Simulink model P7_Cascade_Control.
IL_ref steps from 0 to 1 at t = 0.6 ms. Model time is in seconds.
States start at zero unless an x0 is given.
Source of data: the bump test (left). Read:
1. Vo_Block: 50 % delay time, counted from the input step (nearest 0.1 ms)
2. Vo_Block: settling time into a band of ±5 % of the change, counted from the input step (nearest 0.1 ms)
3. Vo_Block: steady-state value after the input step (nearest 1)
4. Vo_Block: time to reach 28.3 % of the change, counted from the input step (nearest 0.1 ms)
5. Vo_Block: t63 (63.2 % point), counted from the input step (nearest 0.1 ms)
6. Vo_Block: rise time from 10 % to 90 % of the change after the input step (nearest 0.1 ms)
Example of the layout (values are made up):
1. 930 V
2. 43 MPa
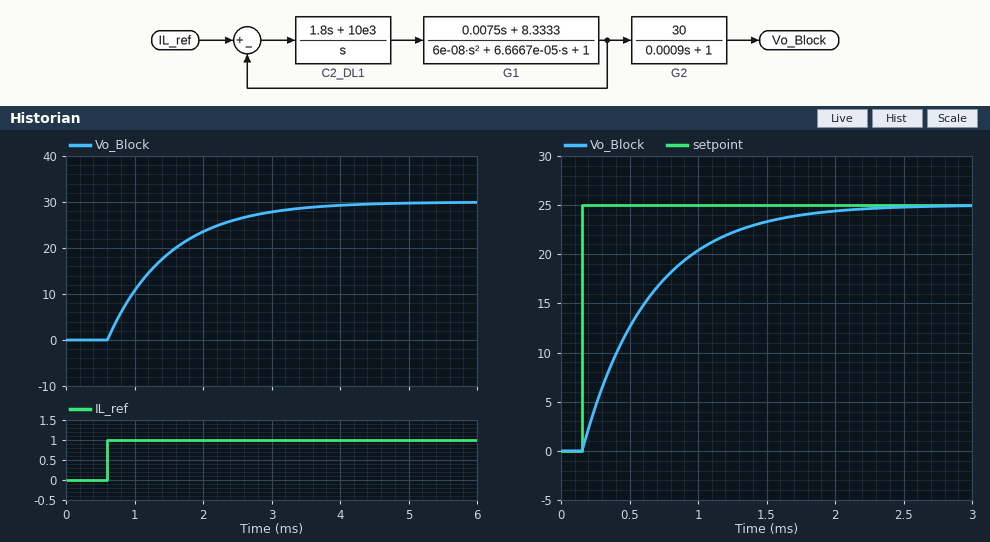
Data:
1. 0.6 ms
2. 2.7 ms
3. 30
4. 0.3 ms
5. 0.9 ms
6. 2.0 ms
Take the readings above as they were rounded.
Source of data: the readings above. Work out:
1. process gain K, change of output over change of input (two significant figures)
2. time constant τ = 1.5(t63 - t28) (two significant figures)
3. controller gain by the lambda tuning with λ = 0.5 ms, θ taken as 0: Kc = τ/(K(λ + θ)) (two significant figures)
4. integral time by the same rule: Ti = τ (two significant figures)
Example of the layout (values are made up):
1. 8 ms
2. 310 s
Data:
1. 30
2. 0.90 ms
3. 0.060
4. 0.90 ms
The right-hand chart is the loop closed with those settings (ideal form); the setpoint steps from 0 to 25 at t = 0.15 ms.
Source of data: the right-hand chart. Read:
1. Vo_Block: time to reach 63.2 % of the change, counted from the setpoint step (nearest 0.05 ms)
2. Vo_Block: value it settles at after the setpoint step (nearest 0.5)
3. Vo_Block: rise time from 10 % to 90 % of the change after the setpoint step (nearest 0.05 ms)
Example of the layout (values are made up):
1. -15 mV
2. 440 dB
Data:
1. 0.50 ms
2. 25.0
3. 1.10 ms
